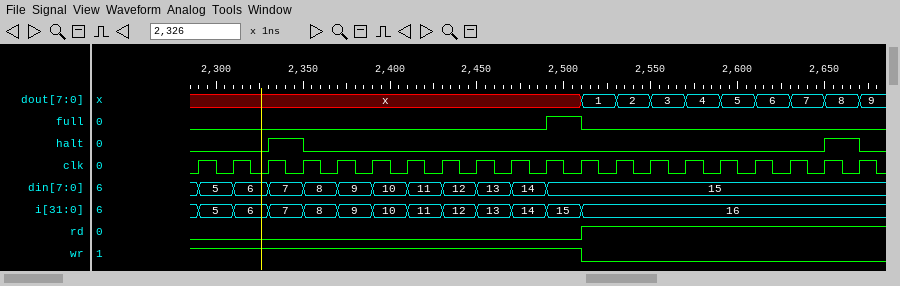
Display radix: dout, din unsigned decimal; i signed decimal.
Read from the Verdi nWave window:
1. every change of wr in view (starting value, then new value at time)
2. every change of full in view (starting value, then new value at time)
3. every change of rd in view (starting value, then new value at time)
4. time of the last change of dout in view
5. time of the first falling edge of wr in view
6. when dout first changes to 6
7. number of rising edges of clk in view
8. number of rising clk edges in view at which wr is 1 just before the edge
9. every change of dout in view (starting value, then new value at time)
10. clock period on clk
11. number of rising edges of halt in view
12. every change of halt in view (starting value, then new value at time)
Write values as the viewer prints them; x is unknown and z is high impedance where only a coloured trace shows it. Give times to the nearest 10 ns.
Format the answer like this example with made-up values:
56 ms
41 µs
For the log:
1, 0 at 2510 ns
0, 1 at 2490 ns, 0 at 2510 ns
0, 1 at 2510 ns
2670 ns
2510 ns
2610 ns
20
12
x, 1 at 2510 ns, 2 at 2530 ns, 3 at 2550 ns, 4 at 2570 ns, 5 at 2590 ns, 6 at 2610 ns, 7 at 2630 ns, 8 at 2650 ns, 9 at 2670 ns
20 ns
2
0, 1 at 2330 ns, 0 at 2350 ns, 1 at 2650 ns, 0 at 2670 ns
